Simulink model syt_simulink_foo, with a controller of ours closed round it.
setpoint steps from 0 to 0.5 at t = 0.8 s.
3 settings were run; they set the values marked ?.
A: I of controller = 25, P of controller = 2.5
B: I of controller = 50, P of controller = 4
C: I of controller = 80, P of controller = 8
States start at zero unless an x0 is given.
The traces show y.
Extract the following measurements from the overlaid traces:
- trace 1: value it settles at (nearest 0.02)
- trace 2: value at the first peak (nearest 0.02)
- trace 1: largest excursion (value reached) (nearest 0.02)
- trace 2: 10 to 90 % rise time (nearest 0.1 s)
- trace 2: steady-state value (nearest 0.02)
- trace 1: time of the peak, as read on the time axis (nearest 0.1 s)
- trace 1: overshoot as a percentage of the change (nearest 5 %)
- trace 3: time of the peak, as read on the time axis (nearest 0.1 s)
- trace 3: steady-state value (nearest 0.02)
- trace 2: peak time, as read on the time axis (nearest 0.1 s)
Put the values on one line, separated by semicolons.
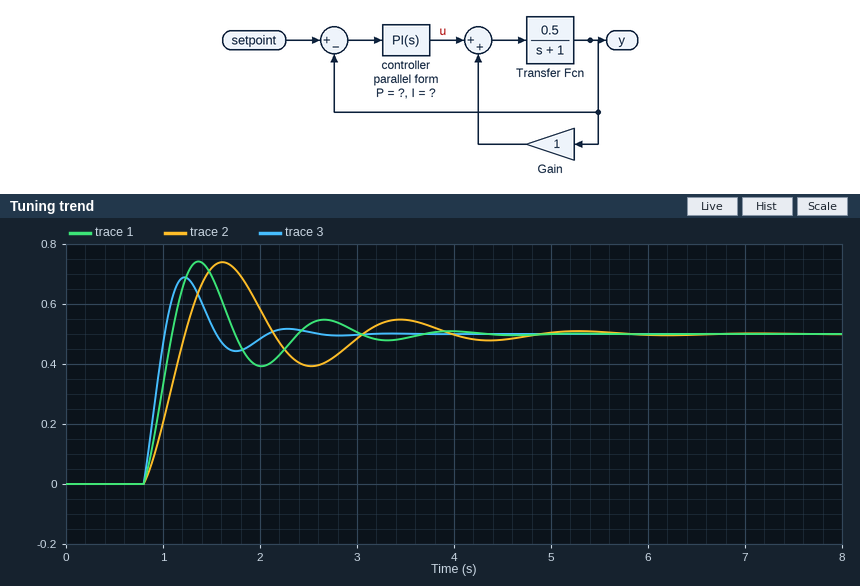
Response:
0.50; 0.74; 0.74; 0.3 s; 0.50; 1.4 s; 50 %; 1.2 s; 0.50; 1.6 s
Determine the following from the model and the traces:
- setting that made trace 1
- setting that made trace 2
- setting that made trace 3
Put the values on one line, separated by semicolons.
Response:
B; A; C
